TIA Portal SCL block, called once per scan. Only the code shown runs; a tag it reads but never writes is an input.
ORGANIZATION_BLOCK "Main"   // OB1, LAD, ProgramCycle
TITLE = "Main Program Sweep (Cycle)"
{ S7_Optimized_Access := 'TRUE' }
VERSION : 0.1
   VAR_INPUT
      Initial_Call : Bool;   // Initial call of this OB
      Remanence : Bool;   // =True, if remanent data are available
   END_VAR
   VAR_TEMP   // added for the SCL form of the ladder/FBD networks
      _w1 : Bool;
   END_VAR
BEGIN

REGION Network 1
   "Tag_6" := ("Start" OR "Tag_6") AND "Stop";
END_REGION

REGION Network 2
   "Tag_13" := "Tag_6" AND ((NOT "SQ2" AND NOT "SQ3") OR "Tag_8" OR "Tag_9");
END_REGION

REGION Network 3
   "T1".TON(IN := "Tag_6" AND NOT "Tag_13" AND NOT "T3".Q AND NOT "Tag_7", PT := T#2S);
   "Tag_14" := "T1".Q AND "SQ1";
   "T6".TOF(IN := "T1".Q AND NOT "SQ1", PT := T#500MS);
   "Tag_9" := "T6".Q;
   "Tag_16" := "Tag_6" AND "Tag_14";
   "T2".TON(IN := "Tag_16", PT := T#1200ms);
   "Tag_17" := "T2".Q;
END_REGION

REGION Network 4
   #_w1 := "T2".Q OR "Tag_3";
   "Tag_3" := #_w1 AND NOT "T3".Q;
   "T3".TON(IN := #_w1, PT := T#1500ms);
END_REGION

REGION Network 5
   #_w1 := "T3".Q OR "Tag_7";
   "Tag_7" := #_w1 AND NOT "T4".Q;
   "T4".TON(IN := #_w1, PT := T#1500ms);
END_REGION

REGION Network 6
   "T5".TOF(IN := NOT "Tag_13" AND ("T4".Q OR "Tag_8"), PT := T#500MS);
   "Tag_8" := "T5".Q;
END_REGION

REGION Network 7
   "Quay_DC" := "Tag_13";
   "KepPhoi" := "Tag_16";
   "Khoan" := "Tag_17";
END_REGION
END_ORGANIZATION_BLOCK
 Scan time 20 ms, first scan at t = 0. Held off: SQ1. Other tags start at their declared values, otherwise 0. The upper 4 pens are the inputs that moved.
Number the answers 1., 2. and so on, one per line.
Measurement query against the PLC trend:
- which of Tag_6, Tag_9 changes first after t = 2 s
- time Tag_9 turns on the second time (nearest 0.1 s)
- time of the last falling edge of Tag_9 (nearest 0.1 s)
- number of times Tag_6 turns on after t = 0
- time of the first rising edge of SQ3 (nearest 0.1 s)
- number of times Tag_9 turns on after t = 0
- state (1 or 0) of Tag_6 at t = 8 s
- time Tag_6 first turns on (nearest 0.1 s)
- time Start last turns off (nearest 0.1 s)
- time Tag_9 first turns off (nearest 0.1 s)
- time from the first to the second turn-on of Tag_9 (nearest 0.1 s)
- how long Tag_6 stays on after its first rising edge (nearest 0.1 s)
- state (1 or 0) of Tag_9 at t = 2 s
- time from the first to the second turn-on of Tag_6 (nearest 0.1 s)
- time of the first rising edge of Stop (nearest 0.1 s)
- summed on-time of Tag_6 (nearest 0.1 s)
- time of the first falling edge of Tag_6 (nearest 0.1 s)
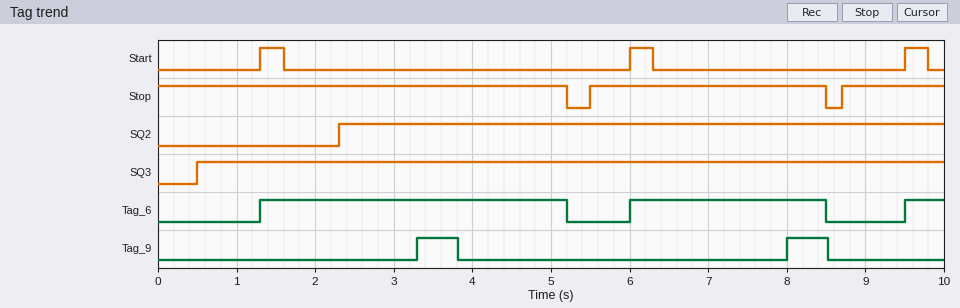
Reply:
1. Tag_9
2. 8.0 s
3. 8.5 s
4. 3
5. 0.5 s
6. 2
7. 1
8. 1.3 s
9. 9.8 s
10. 3.8 s
11. 4.7 s
12. 3.9 s
13. 0
14. 4.7 s
15. 5.5 s
16. 6.9 s
17. 5.2 s
